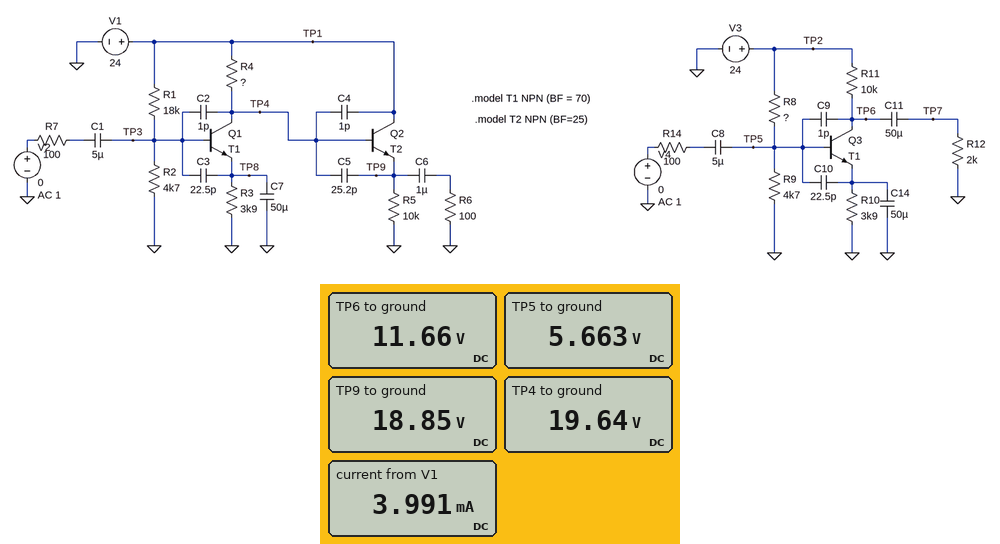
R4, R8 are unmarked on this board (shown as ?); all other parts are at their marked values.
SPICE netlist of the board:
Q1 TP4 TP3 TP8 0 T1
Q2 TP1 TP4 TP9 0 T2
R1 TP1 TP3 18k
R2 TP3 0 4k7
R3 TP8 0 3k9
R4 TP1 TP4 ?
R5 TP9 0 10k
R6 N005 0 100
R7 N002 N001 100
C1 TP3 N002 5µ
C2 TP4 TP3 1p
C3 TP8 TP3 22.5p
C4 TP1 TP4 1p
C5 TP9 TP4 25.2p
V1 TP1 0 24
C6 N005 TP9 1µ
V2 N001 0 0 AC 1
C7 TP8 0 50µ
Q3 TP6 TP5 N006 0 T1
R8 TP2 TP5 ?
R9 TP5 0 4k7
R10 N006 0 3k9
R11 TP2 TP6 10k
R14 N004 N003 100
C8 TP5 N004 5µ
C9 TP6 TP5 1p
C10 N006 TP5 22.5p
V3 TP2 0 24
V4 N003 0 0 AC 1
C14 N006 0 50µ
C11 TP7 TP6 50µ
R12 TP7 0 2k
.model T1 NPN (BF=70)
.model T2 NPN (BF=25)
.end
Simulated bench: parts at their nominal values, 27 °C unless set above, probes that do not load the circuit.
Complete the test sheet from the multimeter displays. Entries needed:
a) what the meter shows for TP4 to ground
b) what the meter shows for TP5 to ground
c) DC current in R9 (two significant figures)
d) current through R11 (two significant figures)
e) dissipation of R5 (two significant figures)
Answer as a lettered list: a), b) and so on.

a) 19.64 V
b) 5.663 V
c) 1.2 mA
d) 1.2 mA
e) 36 mW
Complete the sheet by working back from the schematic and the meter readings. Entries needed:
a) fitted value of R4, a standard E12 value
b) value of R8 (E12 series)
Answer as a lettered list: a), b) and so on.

a) 3.9 kΩ
b) 15 kΩ
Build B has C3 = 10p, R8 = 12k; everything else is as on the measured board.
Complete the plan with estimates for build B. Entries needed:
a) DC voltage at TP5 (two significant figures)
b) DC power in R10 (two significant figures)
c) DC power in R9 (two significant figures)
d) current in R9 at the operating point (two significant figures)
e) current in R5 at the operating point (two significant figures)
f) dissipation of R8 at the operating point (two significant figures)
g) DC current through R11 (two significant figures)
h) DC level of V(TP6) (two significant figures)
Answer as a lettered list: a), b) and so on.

a) 6.7 V
b) 8.9 mW
c) 9.5 mW
d) 1.4 mA
e) 1.9 mA
f) 25 mW
g) 1.5 mA
h) 9.1 V
